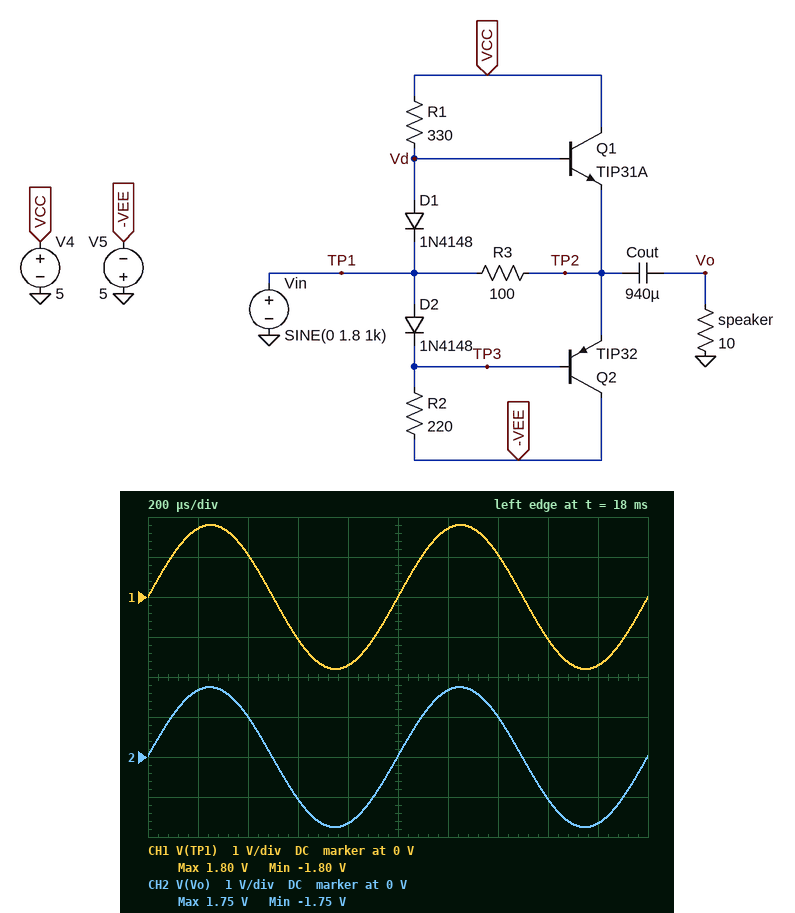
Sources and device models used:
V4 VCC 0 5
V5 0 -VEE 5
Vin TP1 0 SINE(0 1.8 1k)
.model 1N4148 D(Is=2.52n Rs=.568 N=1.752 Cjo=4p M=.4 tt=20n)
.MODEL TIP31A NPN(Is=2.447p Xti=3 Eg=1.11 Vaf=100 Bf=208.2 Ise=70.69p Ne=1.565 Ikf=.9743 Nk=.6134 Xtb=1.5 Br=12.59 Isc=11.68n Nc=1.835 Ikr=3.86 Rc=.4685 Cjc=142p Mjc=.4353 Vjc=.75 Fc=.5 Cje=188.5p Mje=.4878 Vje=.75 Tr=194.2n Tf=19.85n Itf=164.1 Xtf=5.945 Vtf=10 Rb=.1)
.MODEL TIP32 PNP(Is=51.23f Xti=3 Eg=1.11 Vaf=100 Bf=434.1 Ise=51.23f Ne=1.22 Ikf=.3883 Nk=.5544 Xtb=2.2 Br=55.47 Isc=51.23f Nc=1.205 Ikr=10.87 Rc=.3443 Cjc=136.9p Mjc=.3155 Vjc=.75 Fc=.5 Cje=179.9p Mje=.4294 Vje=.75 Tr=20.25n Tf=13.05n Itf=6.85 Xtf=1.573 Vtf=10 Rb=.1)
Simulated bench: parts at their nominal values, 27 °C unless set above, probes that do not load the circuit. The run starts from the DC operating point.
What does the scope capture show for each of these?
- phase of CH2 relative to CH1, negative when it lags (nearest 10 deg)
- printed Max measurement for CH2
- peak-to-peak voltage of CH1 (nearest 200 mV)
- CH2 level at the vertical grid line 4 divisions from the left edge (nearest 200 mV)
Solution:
0 deg
1.75 V
3.6 V
-1.6 V
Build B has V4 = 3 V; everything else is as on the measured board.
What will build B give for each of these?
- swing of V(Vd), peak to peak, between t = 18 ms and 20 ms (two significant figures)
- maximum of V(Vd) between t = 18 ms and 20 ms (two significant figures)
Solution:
3.4 V
2.3 V
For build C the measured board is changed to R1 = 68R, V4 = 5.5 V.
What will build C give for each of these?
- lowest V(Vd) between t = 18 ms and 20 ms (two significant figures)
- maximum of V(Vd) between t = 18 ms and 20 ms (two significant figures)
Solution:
-960 mV
2.6 V
